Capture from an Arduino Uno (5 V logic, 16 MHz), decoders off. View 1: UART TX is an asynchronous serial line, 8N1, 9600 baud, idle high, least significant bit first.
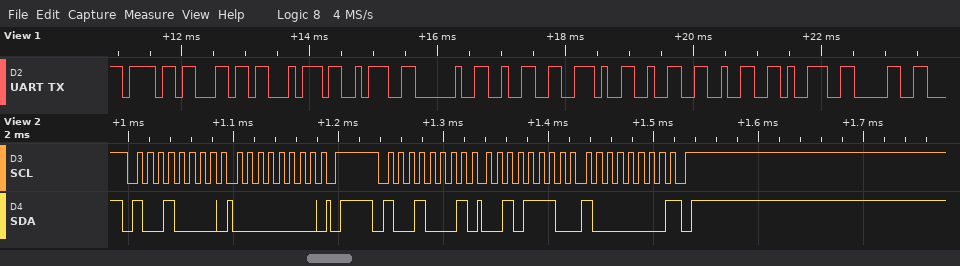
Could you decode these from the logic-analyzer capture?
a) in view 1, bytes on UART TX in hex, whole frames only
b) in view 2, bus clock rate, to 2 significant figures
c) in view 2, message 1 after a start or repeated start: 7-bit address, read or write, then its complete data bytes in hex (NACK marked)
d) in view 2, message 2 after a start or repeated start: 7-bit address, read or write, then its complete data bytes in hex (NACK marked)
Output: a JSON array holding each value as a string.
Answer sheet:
["0x6F 0x6C 0x74 0x3A 0x20 0x32 0x2E 0x32 0x32 0x39 0x30", "100 kHz", "0x48 write: 00", "0x48 read: 2E 80 NACK"]
